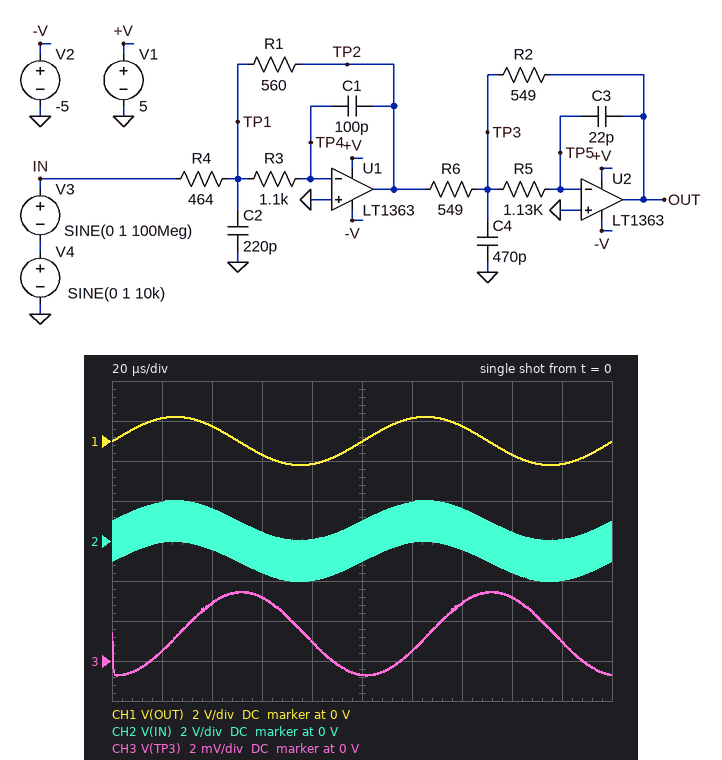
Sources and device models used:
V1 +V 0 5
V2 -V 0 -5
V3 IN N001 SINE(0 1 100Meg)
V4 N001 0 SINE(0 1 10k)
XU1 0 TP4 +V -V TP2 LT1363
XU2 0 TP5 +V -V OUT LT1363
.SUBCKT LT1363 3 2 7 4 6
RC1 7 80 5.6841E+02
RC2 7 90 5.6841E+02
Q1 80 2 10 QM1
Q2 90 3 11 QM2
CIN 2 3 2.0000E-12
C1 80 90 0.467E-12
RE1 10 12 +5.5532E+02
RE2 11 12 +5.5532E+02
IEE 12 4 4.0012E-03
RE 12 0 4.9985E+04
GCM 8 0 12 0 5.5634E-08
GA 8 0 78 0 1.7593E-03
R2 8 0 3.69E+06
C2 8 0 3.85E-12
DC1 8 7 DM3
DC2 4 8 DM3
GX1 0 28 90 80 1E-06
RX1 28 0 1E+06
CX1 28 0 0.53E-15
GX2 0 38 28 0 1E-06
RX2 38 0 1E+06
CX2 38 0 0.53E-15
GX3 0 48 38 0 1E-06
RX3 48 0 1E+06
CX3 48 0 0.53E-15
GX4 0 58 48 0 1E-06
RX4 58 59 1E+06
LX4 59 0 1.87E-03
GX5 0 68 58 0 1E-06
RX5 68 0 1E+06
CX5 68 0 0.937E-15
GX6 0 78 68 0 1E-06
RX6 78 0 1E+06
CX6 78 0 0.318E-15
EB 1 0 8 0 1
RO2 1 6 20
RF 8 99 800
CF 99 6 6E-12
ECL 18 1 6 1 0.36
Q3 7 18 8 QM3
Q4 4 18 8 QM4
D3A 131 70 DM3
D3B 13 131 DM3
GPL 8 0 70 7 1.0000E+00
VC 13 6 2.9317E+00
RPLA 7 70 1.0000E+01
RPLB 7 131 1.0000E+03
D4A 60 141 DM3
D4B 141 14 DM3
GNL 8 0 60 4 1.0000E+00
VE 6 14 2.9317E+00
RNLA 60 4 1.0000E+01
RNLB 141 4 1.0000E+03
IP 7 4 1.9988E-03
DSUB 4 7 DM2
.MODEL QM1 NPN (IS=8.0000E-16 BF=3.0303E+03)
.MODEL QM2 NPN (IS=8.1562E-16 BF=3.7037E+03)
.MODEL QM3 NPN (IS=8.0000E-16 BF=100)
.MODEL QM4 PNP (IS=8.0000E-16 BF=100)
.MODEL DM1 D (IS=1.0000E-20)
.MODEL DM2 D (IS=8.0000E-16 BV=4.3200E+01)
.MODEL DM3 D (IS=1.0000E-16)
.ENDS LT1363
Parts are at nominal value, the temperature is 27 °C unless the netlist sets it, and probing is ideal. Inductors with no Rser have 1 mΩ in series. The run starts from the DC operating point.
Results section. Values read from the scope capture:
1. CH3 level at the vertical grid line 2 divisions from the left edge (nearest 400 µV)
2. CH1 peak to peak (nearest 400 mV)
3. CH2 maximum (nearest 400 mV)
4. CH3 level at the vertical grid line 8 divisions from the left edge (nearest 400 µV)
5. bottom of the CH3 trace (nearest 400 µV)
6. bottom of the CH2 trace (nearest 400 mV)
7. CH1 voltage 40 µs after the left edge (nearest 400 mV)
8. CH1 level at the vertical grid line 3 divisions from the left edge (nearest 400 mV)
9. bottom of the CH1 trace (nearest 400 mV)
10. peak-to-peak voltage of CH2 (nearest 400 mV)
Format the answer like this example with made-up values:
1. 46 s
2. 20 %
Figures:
1. 2.8 mV
2. 2.4 V
3. 2.0 V
4. 3.2 mV
5. -800 µV
6. -2.0 V
7. 800 mV
8. -800 mV
9. -1.2 V
10. 4.0 V
